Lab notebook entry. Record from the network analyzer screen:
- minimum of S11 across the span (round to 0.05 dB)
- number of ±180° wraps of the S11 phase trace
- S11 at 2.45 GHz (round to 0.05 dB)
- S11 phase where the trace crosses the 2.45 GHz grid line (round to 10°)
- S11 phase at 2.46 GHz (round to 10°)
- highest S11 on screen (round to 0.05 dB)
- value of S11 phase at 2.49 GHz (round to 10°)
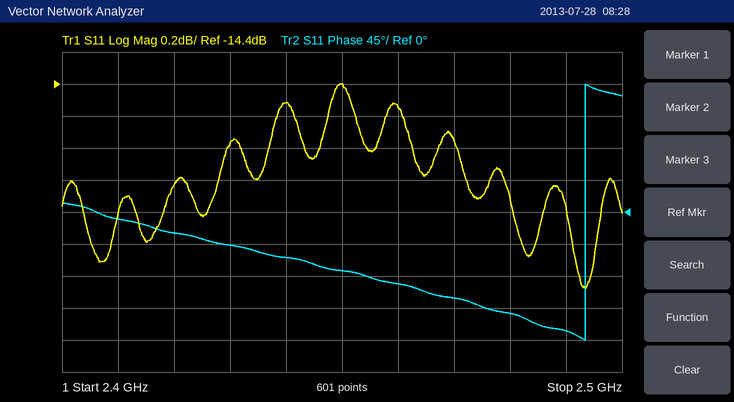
-15.70 dB
1
-14.40 dB
-80°
-100°
-14.40 dB
-170°
